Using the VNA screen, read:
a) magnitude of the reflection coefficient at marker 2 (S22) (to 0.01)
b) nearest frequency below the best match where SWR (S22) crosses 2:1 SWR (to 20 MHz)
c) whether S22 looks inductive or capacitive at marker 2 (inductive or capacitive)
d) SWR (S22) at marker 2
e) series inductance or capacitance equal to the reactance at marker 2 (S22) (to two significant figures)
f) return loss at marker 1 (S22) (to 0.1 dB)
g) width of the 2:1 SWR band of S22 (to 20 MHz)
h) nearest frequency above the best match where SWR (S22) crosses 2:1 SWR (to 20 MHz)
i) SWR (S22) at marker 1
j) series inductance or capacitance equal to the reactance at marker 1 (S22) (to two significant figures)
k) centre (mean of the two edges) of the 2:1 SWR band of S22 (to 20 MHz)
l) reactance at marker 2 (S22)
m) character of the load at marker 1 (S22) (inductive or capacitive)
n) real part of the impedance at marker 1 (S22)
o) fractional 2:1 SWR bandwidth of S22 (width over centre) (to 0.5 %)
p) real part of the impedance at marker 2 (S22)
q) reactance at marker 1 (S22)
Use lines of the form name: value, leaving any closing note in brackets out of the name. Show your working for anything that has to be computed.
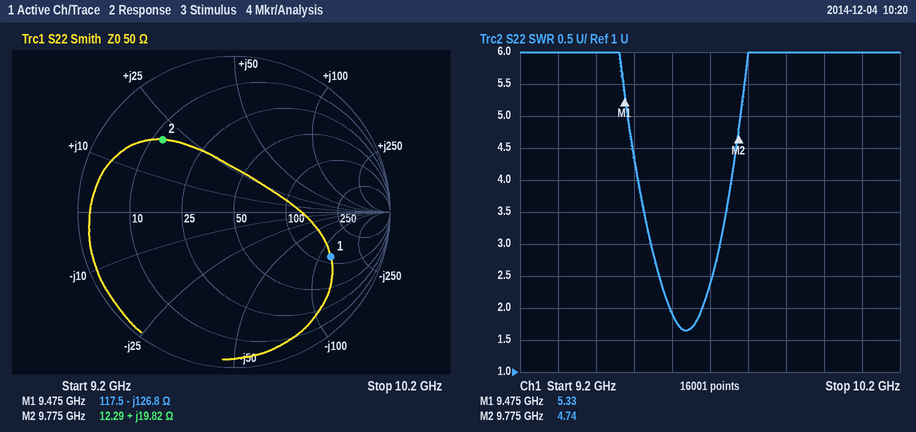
magnitude of the reflection coefficient at marker 2 (S22): 0.65
nearest frequency below the best match where SWR (S22) crosses 2:1 SWR: 9.60 GHz
whether S22 looks inductive or capacitive at marker 2: inductive
SWR (S22) at marker 2: 4.74
series inductance or capacitance equal to the reactance at marker 2 (S22): L = 19.82 Ω/(2π × 9.775 GHz) ≈ 323 pH, so 320 pH to two significant figures
return loss at marker 1 (S22): 3.3 dB
width of the 2:1 SWR band of S22: 9.68 GHz − 9.60 GHz = 80 MHz
nearest frequency above the best match where SWR (S22) crosses 2:1 SWR: 9.68 GHz
SWR (S22) at marker 1: 5.33
series inductance or capacitance equal to the reactance at marker 1 (S22): C = 1/(2π × 9.475 GHz × 126.8 Ω) ≈ 132 fF, so 130 fF to two significant figures
centre (mean of the two edges) of the 2:1 SWR band of S22: 9.64 GHz
reactance at marker 2: +19.82 Ω
character of the load at marker 1 (S22): capacitive
real part of the impedance at marker 1: 117.5 Ω
fractional 2:1 SWR bandwidth of S22 (width over centre): 80 MHz / 9.64 GHz ≈ 0.830 %, so 1.0 % to the nearest 0.5 %
real part of the impedance at marker 2: 12.29 Ω
reactance at marker 1: -126.8 Ω
